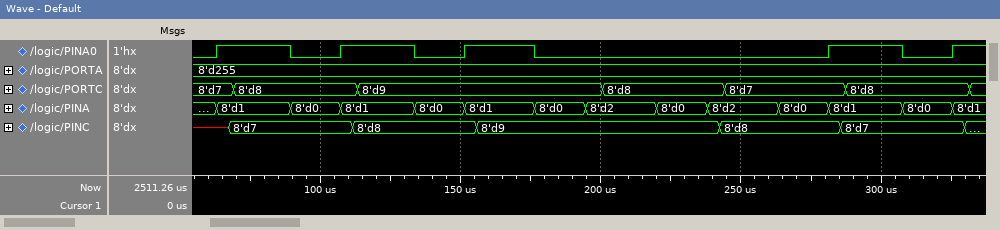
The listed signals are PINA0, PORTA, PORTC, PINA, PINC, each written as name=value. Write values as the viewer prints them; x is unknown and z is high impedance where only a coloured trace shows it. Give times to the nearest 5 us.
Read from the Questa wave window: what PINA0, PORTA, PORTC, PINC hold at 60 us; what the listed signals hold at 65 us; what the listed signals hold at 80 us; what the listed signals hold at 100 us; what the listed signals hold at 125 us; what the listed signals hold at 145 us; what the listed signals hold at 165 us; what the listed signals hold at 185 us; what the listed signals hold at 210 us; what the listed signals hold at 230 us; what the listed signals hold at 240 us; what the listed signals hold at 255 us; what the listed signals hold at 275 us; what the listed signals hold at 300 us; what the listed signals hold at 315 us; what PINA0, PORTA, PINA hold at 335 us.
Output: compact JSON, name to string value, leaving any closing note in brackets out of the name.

{"what PINA0, PORTA, PORTC, PINC hold at 60 us": "PINA0=0, PORTA=8'd255, PORTC=8'd7, PINC=x", "what the listed signals hold at 65 us": "PINA0=1, PORTA=8'd255, PORTC=8'd7, PINA=8'd1, PINC=x", "what the listed signals hold at 80 us": "PINA0=1, PORTA=8'd255, PORTC=8'd8, PINA=8'd1, PINC=8'd7", "what the listed signals hold at 100 us": "PINA0=0, PORTA=8'd255, PORTC=8'd8, PINA=8'd0, PINC=8'd7", "what the listed signals hold at 125 us": "PINA0=1, PORTA=8'd255, PORTC=8'd9, PINA=8'd1, PINC=8'd8", "what the listed signals hold at 145 us": "PINA0=0, PORTA=8'd255, PORTC=8'd9, PINA=8'd0, PINC=8'd8", "what the listed signals hold at 165 us": "PINA0=1, PORTA=8'd255, PORTC=8'd9, PINA=8'd1, PINC=8'd9", "what the listed signals hold at 185 us": "PINA0=0, PORTA=8'd255, PORTC=8'd9, PINA=8'd0, PINC=8'd9", "what the listed signals hold at 210 us": "PINA0=0, PORTA=8'd255, PORTC=8'd8, PINA=8'd2, PINC=8'd9", "what the listed signals hold at 230 us": "PINA0=0, PORTA=8'd255, PORTC=8'd8, PINA=8'd0, PINC=8'd9", "what the listed signals hold at 240 us": "PINA0=0, PORTA=8'd255, PORTC=8'd8, PINA=8'd2, PINC=8'd9", "what the listed signals hold at 255 us": "PINA0=0, PORTA=8'd255, PORTC=8'd7, PINA=8'd2, PINC=8'd8", "what the listed signals hold at 275 us": "PINA0=0, PORTA=8'd255, PORTC=8'd7, PINA=8'd0, PINC=8'd8", "what the listed signals hold at 300 us": "PINA0=1, PORTA=8'd255, PORTC=8'd8, PINA=8'd1, PINC=8'd7", "what the listed signals hold at 315 us": "PINA0=0, PORTA=8'd255, PORTC=8'd8, PINA=8'd0, PINC=8'd7", "what PINA0, PORTA, PINA hold at 335 us": "PINA0=1, PORTA=8'd255, PINA=8'd1"}
